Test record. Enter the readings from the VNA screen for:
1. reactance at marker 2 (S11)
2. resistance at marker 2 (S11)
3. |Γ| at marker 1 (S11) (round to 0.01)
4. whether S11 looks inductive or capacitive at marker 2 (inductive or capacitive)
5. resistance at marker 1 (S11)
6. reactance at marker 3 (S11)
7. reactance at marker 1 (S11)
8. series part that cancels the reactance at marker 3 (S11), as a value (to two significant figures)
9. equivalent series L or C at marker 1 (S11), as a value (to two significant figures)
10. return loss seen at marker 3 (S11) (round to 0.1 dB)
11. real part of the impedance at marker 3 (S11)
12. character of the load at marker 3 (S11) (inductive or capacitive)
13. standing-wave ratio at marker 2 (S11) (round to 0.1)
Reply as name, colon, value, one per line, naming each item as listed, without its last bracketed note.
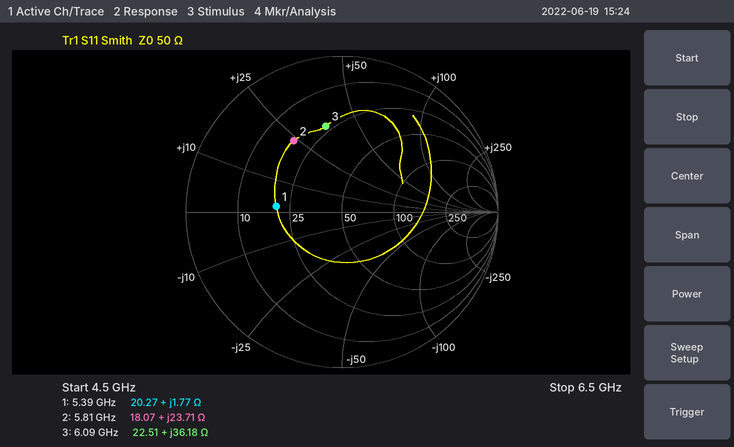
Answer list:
reactance at marker 2: +23.71 Ω
resistance at marker 2: 18.07 Ω
|Γ| at marker 1 (S11): 0.42
whether S11 looks inductive or capacitive at marker 2: inductive
resistance at marker 1: 20.27 Ω
reactance at marker 3: +36.18 Ω
reactance at marker 1: +1.77 Ω
series part that cancels the reactance at marker 3 (S11), as a value: 720 fF
equivalent series L or C at marker 1 (S11), as a value: 52 pH
return loss seen at marker 3 (S11): 5.0 dB
real part of the impedance at marker 3: 22.51 Ω
character of the load at marker 3 (S11): inductive
standing-wave ratio at marker 2 (S11): 3.5
